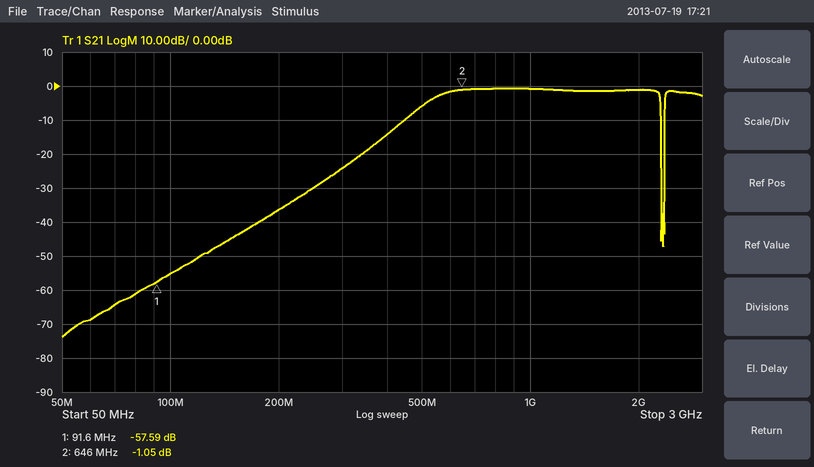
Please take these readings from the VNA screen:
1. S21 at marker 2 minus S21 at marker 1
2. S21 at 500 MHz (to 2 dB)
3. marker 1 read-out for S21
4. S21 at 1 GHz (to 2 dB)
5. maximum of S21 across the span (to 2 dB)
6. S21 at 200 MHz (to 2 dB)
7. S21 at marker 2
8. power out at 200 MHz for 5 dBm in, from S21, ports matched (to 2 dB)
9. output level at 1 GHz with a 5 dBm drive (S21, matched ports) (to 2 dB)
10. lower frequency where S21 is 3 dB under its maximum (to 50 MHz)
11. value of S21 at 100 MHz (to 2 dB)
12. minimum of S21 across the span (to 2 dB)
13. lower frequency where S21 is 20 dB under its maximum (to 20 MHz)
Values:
56.54 dB
-6 dB
-57.59 dB
0 dB
0 dB
-36 dB
-1.05 dB
-32 dBm
4 dBm
550 MHz
-56 dB
-74 dB
340 MHz
